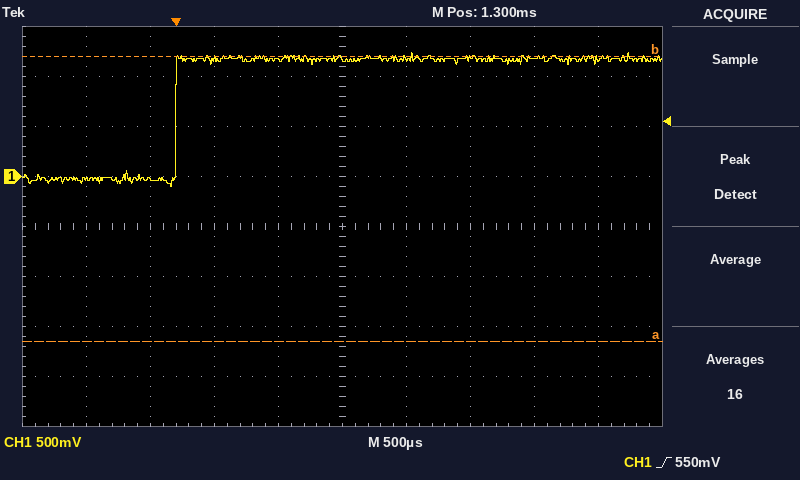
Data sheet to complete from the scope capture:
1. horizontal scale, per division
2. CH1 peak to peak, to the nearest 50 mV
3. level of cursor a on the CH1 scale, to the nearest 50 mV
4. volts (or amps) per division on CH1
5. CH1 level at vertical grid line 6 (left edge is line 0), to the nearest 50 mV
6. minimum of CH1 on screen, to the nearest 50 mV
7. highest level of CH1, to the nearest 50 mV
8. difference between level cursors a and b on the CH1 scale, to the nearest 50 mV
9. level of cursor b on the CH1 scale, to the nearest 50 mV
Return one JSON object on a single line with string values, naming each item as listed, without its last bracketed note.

{"horizontal scale, per division": "500 µs", "CH1 peak to peak, to the nearest 50 mV": "1.35 V", "level of cursor a on the CH1 scale, to the nearest 50 mV": "-1.65 V", "volts (or amps) per division on CH1": "500 mV", "CH1 level at vertical grid line 6 (left edge is line 0), to the nearest 50 mV": "1.20 V", "minimum of CH1 on screen, to the nearest 50 mV": "-100 mV", "highest level of CH1, to the nearest 50 mV": "1.25 V", "difference between level cursors a and b on the CH1 scale, to the nearest 50 mV": "2.85 V", "level of cursor b on the CH1 scale, to the nearest 50 mV": "1.20 V"}
